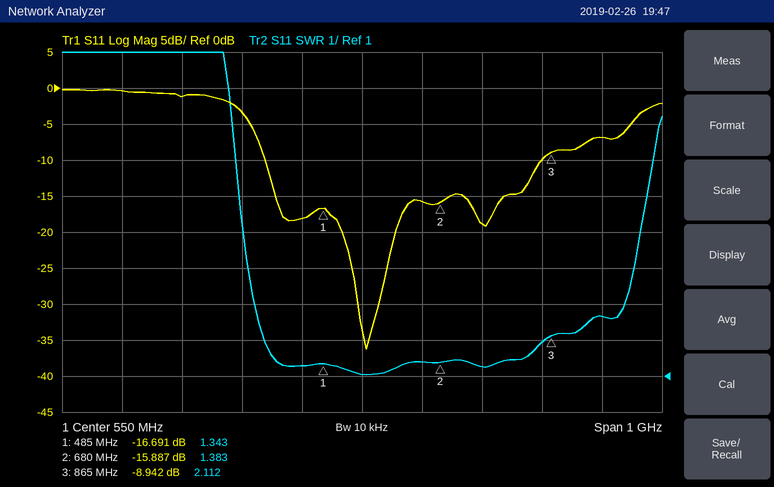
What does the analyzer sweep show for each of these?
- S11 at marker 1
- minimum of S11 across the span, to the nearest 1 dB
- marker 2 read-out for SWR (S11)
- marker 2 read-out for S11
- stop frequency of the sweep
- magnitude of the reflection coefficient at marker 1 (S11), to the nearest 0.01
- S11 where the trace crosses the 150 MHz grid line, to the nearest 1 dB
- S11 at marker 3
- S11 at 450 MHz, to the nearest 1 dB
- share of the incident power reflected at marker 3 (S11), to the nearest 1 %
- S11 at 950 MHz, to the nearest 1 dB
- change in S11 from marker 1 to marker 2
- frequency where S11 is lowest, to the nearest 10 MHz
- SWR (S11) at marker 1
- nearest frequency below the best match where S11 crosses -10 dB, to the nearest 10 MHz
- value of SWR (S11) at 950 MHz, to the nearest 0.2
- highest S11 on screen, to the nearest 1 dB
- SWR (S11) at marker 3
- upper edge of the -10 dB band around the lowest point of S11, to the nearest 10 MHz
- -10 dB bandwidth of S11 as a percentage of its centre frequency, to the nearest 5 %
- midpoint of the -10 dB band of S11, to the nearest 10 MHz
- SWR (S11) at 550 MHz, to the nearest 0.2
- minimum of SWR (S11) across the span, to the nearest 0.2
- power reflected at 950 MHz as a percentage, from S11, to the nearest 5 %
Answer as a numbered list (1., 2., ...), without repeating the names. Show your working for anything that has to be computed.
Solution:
1. -16.691 dB
2. -36 dB
3. 1.383
4. -15.887 dB
5. 1.05 GHz
6. 10^(-16.691/20) ≈ 0.15
7. 0 dB
8. -8.942 dB
9. -18 dB
10. 10^(-8.942/10) ≈ 13 %
11. -7 dB
12. -15.887 − (-16.691) = 0.804 dB
13. 560 MHz
14. 1.343
15. 390 MHz
16. 2.6
17. 0 dB
18. 2.112
19. 850 MHz
20. 460 MHz / 620 MHz ≈ 74.2 %, so 75 % to the nearest 5 %
21. 620 MHz
22. 1.0
23. 1.0
24. 10^(-7/10) ≈ 20 %
